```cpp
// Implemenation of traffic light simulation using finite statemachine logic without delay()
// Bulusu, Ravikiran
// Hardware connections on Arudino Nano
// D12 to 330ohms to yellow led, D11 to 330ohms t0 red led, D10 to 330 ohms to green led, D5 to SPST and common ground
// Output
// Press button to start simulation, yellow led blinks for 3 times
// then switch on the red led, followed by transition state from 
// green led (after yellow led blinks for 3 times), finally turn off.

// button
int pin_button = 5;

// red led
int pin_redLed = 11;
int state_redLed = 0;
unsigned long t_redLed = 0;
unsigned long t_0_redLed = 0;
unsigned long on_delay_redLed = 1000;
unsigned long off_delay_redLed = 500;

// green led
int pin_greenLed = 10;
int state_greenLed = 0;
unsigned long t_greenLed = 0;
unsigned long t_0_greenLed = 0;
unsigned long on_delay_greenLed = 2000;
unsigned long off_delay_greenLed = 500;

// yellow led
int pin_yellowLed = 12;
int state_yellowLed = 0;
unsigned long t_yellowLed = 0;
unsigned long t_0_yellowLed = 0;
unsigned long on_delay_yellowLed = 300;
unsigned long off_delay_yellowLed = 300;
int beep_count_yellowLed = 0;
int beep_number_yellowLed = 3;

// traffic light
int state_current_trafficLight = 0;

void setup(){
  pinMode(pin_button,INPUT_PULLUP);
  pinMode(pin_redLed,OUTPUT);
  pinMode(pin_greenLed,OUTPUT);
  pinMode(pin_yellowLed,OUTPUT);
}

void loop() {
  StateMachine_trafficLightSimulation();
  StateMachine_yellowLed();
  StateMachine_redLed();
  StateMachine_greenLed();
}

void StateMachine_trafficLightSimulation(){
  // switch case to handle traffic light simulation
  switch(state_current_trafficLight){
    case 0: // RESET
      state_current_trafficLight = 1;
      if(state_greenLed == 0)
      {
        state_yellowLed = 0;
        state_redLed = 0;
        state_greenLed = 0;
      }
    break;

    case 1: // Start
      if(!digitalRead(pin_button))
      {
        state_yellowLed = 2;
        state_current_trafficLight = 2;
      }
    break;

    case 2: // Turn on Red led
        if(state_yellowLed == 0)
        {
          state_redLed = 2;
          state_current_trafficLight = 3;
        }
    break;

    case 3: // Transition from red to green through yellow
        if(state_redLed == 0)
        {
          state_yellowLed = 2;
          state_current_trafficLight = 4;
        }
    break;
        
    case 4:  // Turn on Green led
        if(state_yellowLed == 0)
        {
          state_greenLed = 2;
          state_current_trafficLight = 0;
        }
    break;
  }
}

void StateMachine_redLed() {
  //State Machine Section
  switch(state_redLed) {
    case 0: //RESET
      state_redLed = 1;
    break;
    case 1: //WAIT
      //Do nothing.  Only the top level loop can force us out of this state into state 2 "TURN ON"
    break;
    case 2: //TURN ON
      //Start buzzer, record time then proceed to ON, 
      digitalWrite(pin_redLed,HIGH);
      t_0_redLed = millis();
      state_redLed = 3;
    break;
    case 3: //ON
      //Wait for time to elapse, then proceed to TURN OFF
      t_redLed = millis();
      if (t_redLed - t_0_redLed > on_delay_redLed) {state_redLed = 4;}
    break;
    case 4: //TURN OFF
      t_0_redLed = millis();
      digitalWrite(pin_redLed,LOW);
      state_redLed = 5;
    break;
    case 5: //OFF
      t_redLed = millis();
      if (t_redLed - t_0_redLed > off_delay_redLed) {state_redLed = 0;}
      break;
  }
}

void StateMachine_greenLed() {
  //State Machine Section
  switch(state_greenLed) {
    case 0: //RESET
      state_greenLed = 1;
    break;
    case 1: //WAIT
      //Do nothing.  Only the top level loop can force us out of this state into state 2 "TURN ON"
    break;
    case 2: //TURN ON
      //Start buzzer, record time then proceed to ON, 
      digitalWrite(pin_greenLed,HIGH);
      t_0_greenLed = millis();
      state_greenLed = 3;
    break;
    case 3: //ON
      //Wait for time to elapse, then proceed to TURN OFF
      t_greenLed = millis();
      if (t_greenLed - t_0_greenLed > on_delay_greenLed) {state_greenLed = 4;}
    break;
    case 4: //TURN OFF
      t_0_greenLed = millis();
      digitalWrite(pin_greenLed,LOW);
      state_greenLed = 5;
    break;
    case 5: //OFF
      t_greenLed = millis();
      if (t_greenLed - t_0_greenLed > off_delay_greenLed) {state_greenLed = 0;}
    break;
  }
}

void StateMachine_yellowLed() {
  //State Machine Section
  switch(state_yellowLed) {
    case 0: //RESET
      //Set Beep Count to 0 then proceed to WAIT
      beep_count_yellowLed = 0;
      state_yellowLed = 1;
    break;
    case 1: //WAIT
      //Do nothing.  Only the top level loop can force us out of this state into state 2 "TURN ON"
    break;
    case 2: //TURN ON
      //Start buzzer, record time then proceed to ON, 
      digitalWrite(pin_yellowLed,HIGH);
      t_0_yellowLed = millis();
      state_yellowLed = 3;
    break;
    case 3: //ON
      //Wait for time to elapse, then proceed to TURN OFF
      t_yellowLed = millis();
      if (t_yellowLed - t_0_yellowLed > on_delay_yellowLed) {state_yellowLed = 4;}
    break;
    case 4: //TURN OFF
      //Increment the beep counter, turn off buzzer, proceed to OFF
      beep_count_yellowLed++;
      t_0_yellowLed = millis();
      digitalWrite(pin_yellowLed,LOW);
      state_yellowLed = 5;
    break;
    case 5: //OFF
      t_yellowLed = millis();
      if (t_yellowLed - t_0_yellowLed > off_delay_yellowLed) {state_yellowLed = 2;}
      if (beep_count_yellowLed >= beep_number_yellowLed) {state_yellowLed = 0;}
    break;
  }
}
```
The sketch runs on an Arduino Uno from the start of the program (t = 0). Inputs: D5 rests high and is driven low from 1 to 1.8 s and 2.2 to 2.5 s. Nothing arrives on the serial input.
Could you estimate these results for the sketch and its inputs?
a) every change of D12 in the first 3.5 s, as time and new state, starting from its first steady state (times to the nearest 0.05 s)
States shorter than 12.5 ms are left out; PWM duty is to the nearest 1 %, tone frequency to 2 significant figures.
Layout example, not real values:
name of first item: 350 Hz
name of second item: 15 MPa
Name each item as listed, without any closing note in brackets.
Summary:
every change of D12 in the first 3.5 s, as time and new state, starting from its first steady state: 0 s low; 1 s high; 1.3 s low; 1.6 s high; 1.9 s low; 2.2 s high; 2.5 s low
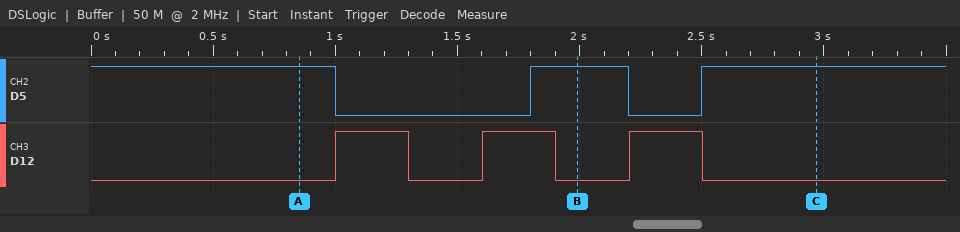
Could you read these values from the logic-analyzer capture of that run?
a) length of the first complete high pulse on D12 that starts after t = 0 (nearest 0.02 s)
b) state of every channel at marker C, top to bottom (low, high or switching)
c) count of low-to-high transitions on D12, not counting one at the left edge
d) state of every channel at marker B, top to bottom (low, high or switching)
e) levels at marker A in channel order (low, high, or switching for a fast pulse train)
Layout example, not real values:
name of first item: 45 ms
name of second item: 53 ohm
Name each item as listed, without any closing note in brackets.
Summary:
length of the first complete high pulse on D12 that starts after t = 0: 0.30 s
state of every channel at marker C, top to bottom: D5 high, D12 low
count of low-to-high transitions on D12, not counting one at the left edge: 3
state of every channel at marker B, top to bottom: D5 high, D12 low
levels at marker A in channel order: D5 high, D12 low
